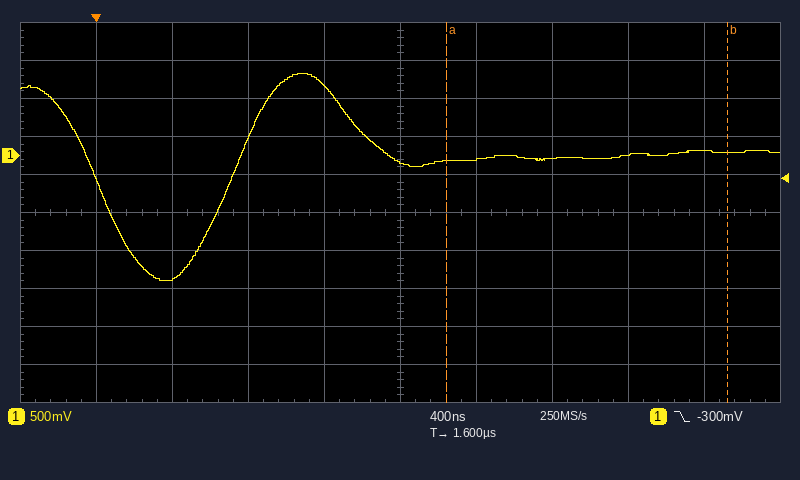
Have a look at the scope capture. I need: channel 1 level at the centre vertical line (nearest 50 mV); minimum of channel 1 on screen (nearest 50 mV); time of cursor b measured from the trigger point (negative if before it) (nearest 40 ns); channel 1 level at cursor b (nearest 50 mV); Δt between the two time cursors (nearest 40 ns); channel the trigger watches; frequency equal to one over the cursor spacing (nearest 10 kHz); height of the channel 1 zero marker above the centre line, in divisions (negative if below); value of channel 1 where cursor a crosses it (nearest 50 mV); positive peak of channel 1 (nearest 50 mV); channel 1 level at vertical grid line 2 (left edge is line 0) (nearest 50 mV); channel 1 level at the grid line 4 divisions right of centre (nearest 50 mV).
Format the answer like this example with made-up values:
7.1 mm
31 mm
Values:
-100 mV
-1.65 V
+3.32 µs
50 mV
1.48 µs
channel 1
680 kHz
+1.5 div
-50 mV
1.10 V
-1.60 V
50 mV
